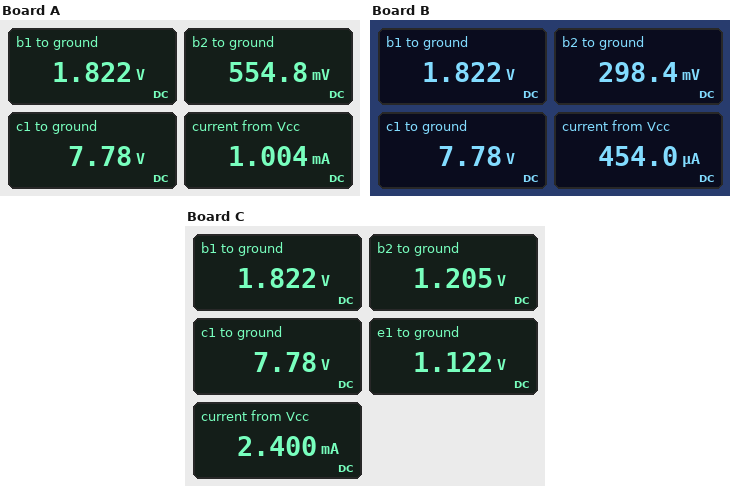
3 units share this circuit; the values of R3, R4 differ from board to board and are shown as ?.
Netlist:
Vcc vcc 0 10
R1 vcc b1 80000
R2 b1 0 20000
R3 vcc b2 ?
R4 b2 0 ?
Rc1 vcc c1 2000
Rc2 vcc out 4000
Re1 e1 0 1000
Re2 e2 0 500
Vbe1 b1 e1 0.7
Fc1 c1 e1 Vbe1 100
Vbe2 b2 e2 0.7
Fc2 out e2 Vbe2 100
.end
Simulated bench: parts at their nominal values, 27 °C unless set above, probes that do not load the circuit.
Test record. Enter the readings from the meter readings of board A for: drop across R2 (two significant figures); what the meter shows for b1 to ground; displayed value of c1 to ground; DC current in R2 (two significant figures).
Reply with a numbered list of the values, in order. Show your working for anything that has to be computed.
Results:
1. 1.822 V = 1.8 V
2. 1.822 V
3. 7.78 V
4. (1.822 V) / 20 kΩ = 91 µA
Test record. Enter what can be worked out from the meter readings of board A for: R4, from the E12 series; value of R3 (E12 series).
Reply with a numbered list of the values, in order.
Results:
1. 6.8 kΩ
2. 120 kΩ
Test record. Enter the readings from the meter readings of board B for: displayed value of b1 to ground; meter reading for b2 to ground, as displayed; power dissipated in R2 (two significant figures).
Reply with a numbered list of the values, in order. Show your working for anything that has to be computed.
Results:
1. 1.822 V
2. 298.4 mV
3. (1.822 V)^2 / 20 kΩ = 170 µW
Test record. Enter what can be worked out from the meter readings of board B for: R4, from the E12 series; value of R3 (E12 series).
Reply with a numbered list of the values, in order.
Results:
1. 6.8 kΩ
2. 270 kΩ
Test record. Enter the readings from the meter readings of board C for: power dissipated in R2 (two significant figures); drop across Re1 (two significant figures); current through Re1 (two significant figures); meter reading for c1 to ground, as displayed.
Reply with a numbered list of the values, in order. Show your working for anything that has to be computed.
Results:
1. (1.822 V)^2 / 20 kΩ = 170 µW
2. 1.122 V = 1.1 V
3. (1.122 V) / 1 kΩ = 1.1 mA
4. 7.78 V
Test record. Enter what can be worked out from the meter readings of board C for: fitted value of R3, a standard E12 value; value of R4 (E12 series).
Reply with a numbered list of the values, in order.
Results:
1. 47 kΩ
2. 6.8 kΩ
